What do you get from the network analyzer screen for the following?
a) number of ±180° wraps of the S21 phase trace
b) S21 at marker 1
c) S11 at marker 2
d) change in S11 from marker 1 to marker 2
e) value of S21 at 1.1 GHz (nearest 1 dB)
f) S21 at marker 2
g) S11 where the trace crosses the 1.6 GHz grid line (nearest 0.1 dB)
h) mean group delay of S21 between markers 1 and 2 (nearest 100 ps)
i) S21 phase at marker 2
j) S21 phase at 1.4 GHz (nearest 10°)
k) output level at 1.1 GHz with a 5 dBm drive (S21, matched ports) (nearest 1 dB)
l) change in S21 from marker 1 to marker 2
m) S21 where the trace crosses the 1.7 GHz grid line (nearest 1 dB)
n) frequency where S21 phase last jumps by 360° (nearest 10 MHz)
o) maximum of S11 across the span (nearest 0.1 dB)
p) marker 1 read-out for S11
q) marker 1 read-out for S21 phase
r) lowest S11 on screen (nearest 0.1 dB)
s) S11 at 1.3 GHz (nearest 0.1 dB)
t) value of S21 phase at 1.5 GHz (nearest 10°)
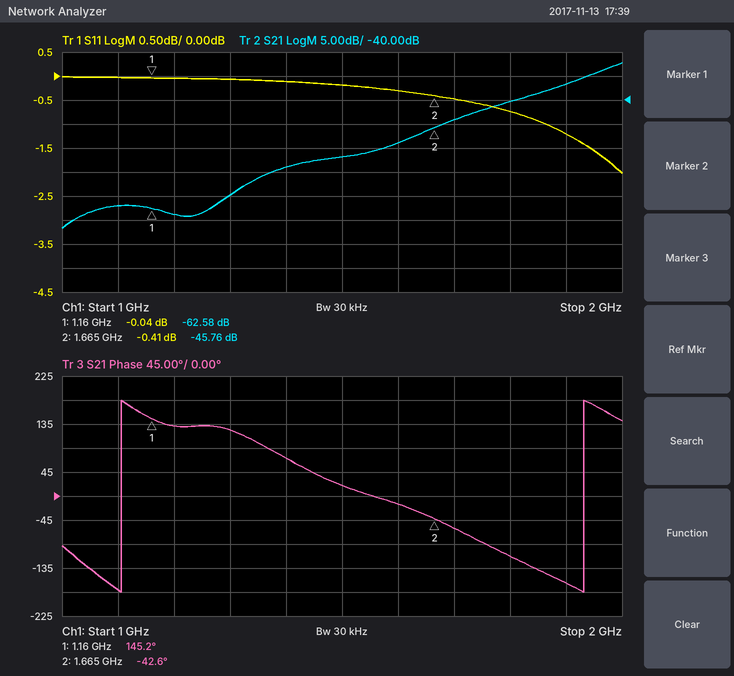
2
-62.58 dB
-0.41 dB
-0.37 dB
-62 dB
-45.76 dB
-0.3 dB
1.0 ns
-42.6°
70°
-57 dBm
16.82 dB
-44 dB
1.93 GHz
0.0 dB
-0.04 dB
145.2°
-2.0 dB
-0.1 dB
20°
